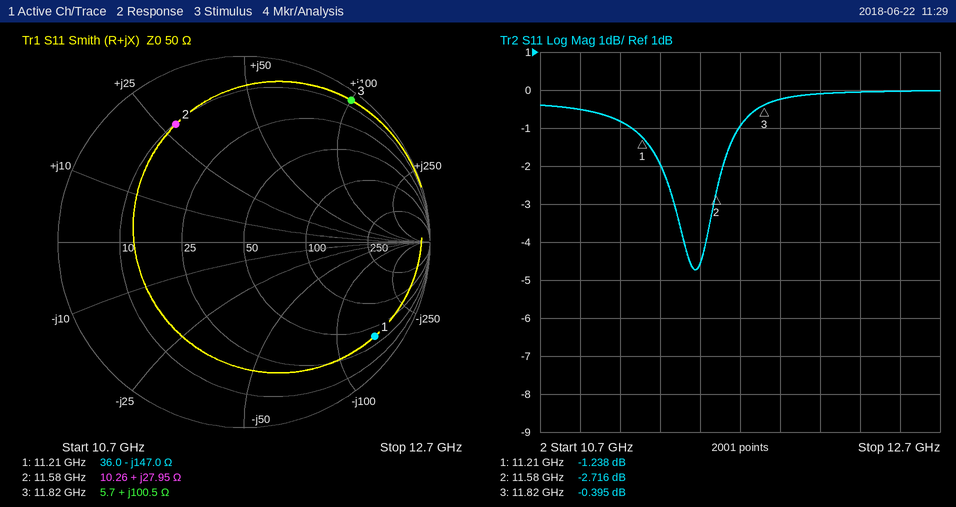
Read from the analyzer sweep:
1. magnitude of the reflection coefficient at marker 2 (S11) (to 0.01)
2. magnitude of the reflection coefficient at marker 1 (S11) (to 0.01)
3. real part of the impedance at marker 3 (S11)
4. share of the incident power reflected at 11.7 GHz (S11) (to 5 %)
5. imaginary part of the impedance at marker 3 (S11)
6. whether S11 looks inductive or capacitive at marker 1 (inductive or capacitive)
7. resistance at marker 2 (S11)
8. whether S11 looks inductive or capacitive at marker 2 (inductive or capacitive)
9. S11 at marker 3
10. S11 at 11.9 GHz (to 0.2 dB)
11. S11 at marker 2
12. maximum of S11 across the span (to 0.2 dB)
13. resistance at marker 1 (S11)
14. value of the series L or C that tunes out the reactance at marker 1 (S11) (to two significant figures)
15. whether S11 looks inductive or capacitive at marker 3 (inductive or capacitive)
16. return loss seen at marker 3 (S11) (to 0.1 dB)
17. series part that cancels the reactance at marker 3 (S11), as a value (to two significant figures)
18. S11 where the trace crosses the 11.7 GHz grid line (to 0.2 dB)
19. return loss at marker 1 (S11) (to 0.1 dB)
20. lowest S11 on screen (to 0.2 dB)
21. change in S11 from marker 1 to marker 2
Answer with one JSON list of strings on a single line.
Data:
["0.73", "0.87", "5.7 Ω", "80 %", "+100.5 Ω", "capacitive", "10.26 Ω", "inductive", "-0.395 dB", "-0.2 dB", "-2.716 dB", "0.0 dB", "36.0 Ω", "2.1 nH", "inductive", "0.4 dB", "130 fF", "-1.0 dB", "1.2 dB", "-4.8 dB", "-1.478 dB"]
